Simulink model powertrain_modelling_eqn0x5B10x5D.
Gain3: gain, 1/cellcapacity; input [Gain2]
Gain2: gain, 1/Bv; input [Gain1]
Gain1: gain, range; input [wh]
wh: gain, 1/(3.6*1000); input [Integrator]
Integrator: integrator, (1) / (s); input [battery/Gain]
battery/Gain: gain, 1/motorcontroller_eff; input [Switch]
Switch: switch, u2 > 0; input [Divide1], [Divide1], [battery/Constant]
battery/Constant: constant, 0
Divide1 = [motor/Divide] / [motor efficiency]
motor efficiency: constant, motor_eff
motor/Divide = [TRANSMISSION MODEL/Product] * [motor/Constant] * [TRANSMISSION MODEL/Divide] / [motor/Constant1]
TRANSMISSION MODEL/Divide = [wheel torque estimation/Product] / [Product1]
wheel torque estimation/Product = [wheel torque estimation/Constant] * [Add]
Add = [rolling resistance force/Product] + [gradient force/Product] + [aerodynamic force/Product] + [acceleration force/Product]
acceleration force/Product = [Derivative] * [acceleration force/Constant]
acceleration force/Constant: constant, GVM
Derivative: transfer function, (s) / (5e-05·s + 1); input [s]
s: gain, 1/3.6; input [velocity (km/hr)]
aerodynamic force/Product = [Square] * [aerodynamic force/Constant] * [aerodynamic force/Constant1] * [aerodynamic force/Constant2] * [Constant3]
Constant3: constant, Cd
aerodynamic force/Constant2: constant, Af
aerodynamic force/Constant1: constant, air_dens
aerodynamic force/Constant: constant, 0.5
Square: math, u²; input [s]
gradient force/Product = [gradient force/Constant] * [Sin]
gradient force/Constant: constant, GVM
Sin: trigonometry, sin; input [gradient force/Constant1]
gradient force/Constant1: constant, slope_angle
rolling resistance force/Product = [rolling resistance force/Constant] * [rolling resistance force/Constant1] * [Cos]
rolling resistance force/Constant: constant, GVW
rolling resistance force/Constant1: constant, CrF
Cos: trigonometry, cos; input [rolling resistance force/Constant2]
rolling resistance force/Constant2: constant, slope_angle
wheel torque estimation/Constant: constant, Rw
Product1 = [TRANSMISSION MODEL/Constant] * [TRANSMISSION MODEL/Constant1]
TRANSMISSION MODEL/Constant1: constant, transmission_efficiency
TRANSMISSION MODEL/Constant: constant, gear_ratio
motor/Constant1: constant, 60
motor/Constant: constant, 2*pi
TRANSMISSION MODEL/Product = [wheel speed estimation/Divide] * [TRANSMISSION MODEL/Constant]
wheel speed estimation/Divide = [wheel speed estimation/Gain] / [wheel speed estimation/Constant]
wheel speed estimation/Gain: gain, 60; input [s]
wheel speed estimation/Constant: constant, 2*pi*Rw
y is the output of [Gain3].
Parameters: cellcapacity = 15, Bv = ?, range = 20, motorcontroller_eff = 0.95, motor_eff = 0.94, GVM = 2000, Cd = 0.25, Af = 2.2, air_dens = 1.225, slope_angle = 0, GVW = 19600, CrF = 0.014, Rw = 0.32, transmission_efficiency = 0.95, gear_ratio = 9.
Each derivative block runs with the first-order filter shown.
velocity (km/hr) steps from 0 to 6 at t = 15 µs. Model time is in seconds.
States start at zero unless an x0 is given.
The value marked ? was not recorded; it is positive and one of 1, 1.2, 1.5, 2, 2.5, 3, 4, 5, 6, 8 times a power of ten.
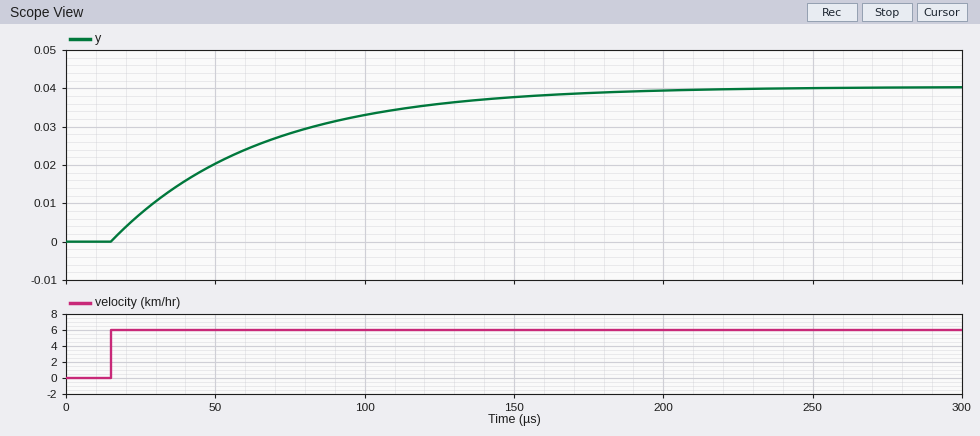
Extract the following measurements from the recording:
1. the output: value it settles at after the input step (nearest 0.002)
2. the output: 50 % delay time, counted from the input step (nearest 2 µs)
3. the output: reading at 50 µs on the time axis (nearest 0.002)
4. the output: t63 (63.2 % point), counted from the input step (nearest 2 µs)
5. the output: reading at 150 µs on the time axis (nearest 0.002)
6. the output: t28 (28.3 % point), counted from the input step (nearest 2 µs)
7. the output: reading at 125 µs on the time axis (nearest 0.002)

0.040
34 µs
0.020
50 µs
0.038
16 µs
0.036
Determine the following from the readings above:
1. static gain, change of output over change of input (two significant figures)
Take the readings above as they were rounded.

0.0067
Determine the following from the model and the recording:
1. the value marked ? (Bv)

60
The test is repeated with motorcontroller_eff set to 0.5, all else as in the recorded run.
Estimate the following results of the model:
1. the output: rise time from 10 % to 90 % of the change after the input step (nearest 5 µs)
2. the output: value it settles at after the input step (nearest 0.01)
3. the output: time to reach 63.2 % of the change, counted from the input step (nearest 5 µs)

110 µs
0.08
50 µs
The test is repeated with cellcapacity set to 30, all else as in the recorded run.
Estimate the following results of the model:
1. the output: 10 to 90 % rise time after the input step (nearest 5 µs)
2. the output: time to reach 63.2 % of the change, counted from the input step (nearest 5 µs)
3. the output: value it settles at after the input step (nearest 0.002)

110 µs
50 µs
0.020
